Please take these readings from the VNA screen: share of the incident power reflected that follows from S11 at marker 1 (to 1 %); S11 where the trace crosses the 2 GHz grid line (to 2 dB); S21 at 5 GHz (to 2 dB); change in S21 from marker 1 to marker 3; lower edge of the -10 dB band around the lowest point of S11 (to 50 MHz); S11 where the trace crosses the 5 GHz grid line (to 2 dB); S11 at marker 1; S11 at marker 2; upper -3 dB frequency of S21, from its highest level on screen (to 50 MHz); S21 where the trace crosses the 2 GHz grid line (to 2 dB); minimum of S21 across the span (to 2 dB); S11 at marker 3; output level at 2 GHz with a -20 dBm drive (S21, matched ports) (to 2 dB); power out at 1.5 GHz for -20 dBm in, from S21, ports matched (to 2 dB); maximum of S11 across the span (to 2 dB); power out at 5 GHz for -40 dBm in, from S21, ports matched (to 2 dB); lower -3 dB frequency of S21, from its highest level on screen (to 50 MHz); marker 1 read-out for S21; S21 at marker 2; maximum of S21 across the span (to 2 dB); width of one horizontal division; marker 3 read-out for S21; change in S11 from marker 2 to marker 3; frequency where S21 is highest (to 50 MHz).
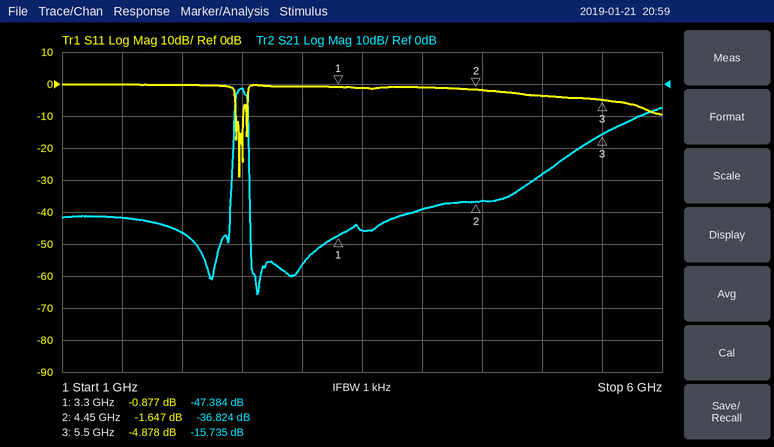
82 %
0 dB
-28 dB
31.649 dB
2.45 GHz
-4 dB
-0.877 dB
-1.647 dB
2.55 GHz
-46 dB
-66 dB
-4.878 dB
-66 dBm
-62 dBm
0 dB
-68 dBm
2.45 GHz
-47.384 dB
-36.824 dB
-2 dB
500 MHz
-15.735 dB
-3.231 dB
2.50 GHz
